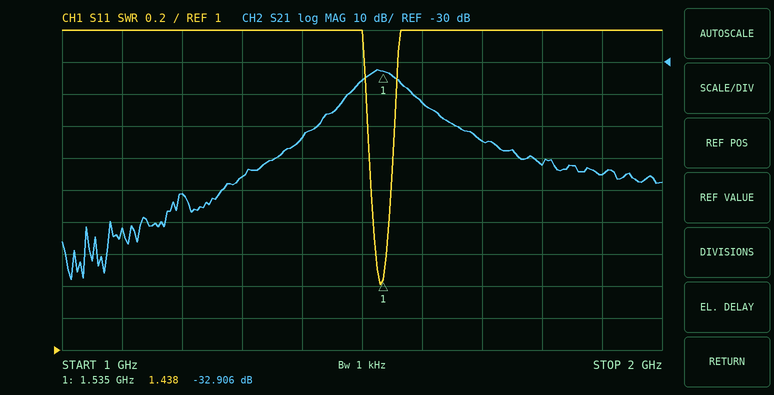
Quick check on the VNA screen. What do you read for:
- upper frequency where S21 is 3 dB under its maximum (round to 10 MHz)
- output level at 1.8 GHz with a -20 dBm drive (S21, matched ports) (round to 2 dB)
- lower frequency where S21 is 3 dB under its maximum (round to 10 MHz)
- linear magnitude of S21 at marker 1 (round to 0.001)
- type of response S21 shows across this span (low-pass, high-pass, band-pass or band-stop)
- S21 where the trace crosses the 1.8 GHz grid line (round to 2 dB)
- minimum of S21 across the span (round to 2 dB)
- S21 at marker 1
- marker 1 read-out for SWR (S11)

1.56 GHz
-82 dBm
1.50 GHz
0.023
band-pass
-62 dB
-98 dB
-32.906 dB
1.438
